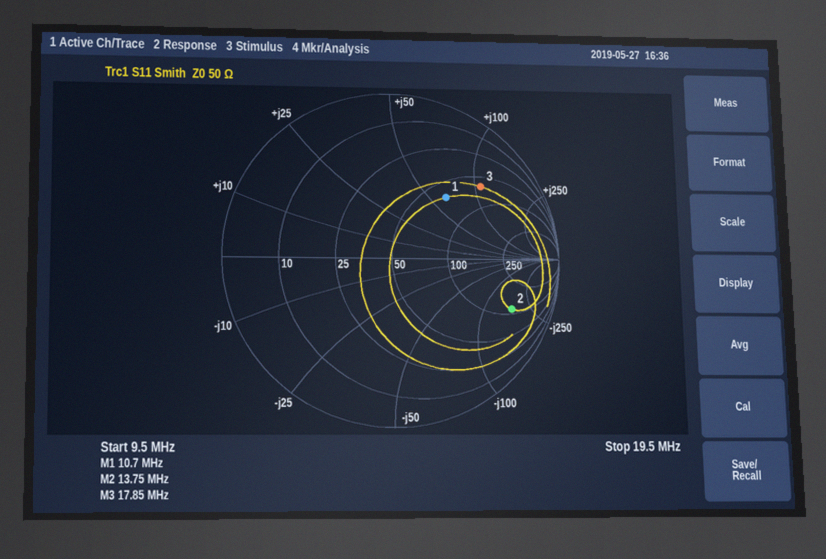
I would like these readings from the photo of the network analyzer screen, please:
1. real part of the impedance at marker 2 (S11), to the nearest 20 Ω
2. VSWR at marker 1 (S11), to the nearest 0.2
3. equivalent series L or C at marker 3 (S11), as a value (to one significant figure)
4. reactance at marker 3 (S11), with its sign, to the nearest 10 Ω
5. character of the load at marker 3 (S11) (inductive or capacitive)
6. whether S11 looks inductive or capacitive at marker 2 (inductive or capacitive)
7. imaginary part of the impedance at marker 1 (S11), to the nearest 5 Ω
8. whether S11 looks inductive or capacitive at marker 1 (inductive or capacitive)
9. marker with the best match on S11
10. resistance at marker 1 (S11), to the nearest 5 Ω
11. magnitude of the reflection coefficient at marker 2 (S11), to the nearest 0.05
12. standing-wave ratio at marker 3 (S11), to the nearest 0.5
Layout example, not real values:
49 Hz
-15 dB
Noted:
120 Ω
3.0
1.0 µH
+110 Ω
inductive
capacitive
+65 Ω
inductive
marker 1
65 Ω
0.75
5.5
